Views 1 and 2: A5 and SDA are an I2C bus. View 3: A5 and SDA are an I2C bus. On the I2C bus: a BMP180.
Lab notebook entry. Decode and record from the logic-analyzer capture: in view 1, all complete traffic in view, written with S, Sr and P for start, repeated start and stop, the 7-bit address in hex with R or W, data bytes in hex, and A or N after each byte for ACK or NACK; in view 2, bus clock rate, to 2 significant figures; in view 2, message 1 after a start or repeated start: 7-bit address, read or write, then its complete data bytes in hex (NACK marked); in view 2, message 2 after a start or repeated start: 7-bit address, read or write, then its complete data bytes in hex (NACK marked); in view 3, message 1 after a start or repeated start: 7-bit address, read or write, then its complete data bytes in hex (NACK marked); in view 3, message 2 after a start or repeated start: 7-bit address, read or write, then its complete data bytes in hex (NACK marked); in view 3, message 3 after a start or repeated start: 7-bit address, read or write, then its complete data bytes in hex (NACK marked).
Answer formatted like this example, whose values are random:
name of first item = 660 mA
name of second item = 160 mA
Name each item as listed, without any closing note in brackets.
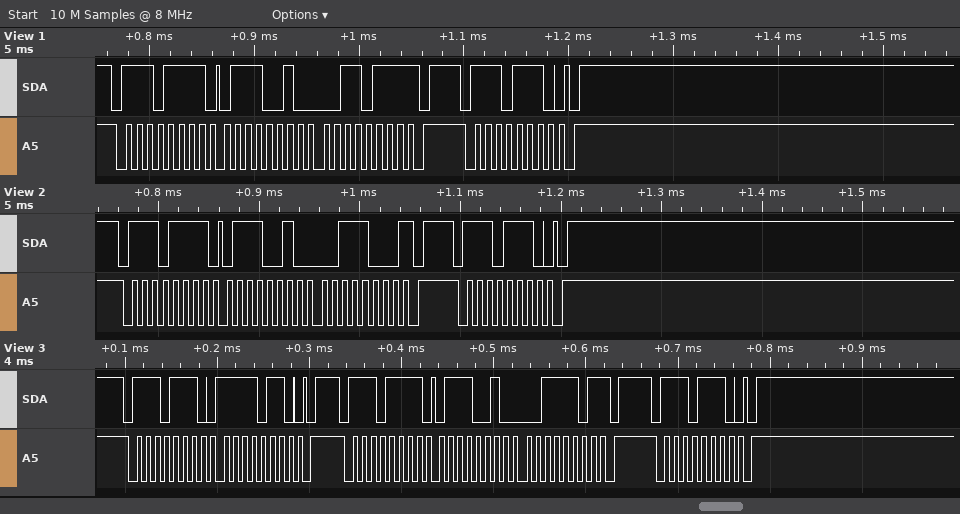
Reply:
in view 1, all complete traffic in view, written with S, Sr and P for start, repeated start and stop, the 7-bit address in hex with R or W, data bytes in hex, and A or N after each byte for ACK or NACK = S 77R A 72 A 37 N P S 77W A P
in view 2, bus clock rate, to 2 significant figures = 100 kHz
in view 2, message 1 after a start or repeated start: 7-bit address, read or write, then its complete data bytes in hex = 0x77 read: 72 38 NACK
in view 2, message 2 after a start or repeated start: 7-bit address, read or write, then its complete data bytes in hex = 0x77 write
in view 3, message 1 after a start or repeated start: 7-bit address, read or write, then its complete data bytes in hex = 0x77 write: F6
in view 3, message 2 after a start or repeated start: 7-bit address, read or write, then its complete data bytes in hex = 0x77 read: 72 3D NACK
in view 3, message 3 after a start or repeated start: 7-bit address, read or write, then its complete data bytes in hex = 0x77 write
